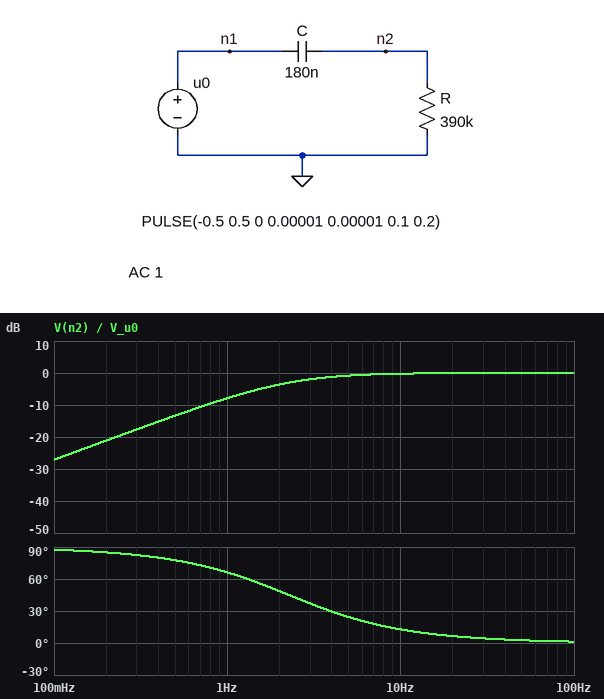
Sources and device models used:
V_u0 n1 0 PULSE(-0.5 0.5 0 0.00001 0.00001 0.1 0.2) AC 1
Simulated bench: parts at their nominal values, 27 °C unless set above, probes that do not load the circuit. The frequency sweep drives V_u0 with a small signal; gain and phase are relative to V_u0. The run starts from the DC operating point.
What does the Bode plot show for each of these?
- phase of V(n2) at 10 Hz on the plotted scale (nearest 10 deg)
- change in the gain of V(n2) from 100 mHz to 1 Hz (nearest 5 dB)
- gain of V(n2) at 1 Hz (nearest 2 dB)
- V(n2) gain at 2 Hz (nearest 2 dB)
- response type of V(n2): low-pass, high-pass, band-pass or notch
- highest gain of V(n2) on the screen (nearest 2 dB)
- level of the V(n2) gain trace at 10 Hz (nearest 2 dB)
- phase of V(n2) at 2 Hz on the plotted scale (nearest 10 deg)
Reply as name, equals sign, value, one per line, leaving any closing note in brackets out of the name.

phase of V(n2) at 10 Hz on the plotted scale = 10 deg
change in the gain of V(n2) from 100 mHz to 1 Hz = 20 dB
gain of V(n2) at 1 Hz = -8 dB
V(n2) gain at 2 Hz = -4 dB
response type of V(n2): low-pass, high-pass, band-pass or notch = high-pass
highest gain of V(n2) on the screen = 0 dB
level of the V(n2) gain trace at 10 Hz = 0 dB
phase of V(n2) at 2 Hz on the plotted scale = 50 deg
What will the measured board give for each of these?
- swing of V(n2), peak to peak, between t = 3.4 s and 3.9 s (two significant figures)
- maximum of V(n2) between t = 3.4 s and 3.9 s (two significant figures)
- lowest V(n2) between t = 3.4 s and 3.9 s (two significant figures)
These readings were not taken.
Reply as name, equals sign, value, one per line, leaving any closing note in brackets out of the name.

swing of V(n2), peak to peak, between t = 3.4 s and 3.9 s = 1.6 V
maximum of V(n2) between t = 3.4 s and 3.9 s = 810 mV
lowest V(n2) between t = 3.4 s and 3.9 s = -810 mV
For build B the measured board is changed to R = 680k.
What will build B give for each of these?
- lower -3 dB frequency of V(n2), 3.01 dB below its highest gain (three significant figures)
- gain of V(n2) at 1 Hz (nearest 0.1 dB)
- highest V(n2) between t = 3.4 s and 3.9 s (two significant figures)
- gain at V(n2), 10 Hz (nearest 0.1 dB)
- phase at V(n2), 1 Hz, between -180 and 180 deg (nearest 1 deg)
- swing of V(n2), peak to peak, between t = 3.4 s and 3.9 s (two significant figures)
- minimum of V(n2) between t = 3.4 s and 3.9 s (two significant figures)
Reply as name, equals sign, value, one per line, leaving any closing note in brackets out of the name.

lower -3 dB frequency of V(n2), 3.01 dB below its highest gain = 1.30 Hz
gain of V(n2) at 1 Hz = -4.3 dB
highest V(n2) between t = 3.4 s and 3.9 s = 690 mV
gain at V(n2), 10 Hz = -0.1 dB
phase at V(n2), 1 Hz, between -180 and 180 deg = 52 deg
swing of V(n2), peak to peak, between t = 3.4 s and 3.9 s = 1.4 V
minimum of V(n2) between t = 3.4 s and 3.9 s = -690 mV
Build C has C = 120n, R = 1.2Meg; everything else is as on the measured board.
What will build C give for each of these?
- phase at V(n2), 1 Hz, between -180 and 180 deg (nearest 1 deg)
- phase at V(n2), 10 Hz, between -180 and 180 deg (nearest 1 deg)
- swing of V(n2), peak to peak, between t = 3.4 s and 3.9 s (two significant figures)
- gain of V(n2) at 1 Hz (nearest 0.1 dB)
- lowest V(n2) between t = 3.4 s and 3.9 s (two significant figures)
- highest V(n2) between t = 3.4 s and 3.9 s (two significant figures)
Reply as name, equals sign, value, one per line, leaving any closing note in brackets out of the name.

phase at V(n2), 1 Hz, between -180 and 180 deg = 48 deg
phase at V(n2), 10 Hz, between -180 and 180 deg = 6 deg
swing of V(n2), peak to peak, between t = 3.4 s and 3.9 s = 1.3 V
gain of V(n2) at 1 Hz = -3.5 dB
lowest V(n2) between t = 3.4 s and 3.9 s = -670 mV
highest V(n2) between t = 3.4 s and 3.9 s = 670 mV
